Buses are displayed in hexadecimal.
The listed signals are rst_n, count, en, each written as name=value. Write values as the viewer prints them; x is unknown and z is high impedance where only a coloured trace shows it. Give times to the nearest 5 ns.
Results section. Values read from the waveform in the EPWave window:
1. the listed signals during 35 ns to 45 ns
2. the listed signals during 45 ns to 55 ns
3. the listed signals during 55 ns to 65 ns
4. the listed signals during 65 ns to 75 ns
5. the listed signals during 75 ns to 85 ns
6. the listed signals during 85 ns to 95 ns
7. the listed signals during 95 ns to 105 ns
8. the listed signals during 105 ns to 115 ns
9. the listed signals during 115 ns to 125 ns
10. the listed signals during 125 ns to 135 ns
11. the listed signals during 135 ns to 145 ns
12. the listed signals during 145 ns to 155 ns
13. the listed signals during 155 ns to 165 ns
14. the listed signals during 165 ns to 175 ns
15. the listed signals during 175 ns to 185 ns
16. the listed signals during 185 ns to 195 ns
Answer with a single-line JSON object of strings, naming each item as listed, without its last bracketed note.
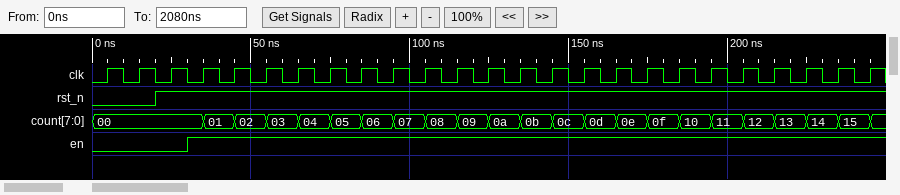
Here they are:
{"the listed signals during 35 ns to 45 ns": "rst_n=1, count=01, en=1", "the listed signals during 45 ns to 55 ns": "rst_n=1, count=02, en=1", "the listed signals during 55 ns to 65 ns": "rst_n=1, count=03, en=1", "the listed signals during 65 ns to 75 ns": "rst_n=1, count=04, en=1", "the listed signals during 75 ns to 85 ns": "rst_n=1, count=05, en=1", "the listed signals during 85 ns to 95 ns": "rst_n=1, count=06, en=1", "the listed signals during 95 ns to 105 ns": "rst_n=1, count=07, en=1", "the listed signals during 105 ns to 115 ns": "rst_n=1, count=08, en=1", "the listed signals during 115 ns to 125 ns": "rst_n=1, count=09, en=1", "the listed signals during 125 ns to 135 ns": "rst_n=1, count=0a, en=1", "the listed signals during 135 ns to 145 ns": "rst_n=1, count=0b, en=1", "the listed signals during 145 ns to 155 ns": "rst_n=1, count=0c, en=1", "the listed signals during 155 ns to 165 ns": "rst_n=1, count=0d, en=1", "the listed signals during 165 ns to 175 ns": "rst_n=1, count=0e, en=1", "the listed signals during 175 ns to 185 ns": "rst_n=1, count=0f, en=1", "the listed signals during 185 ns to 195 ns": "rst_n=1, count=10, en=1"}
